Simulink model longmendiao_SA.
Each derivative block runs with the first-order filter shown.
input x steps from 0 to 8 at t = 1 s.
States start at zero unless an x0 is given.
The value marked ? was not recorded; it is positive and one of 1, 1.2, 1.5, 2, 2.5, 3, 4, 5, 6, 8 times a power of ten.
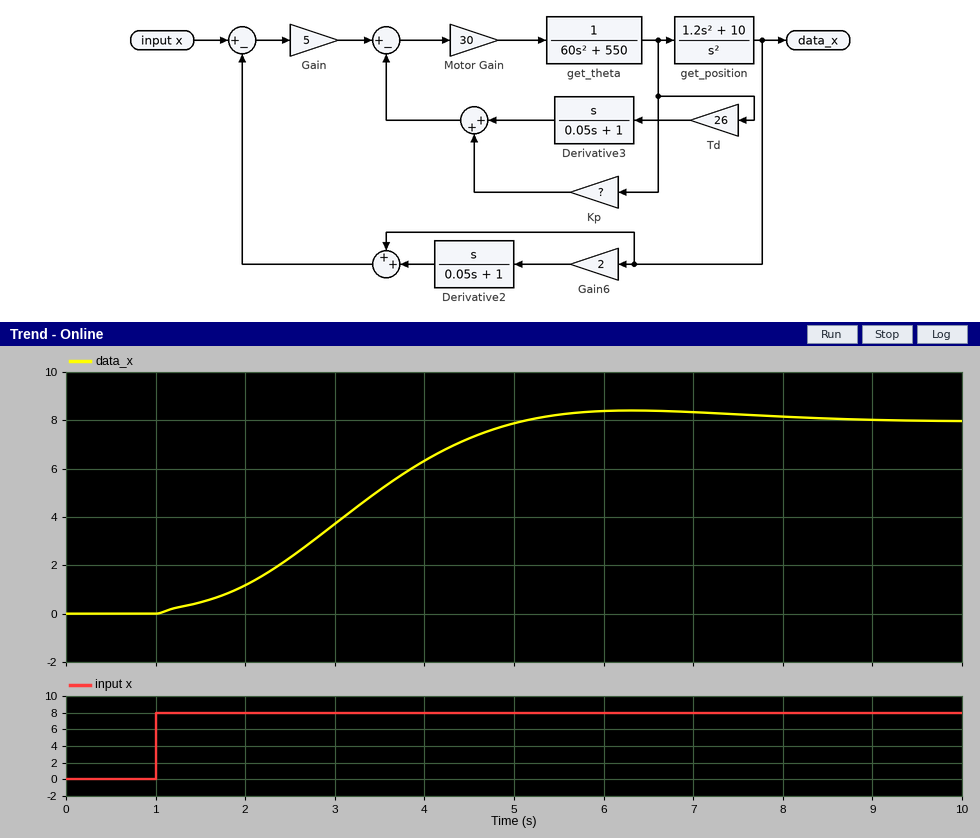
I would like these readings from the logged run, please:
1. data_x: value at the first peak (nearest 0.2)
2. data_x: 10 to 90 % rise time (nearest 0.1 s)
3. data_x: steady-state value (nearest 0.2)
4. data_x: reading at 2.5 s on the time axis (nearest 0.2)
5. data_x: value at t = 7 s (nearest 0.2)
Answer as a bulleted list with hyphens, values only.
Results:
- 8.4
- 2.7 s
- 8.0
- 2.4
- 8.4
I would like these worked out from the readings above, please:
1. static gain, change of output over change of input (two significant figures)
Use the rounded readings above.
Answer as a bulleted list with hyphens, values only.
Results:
- 1.0
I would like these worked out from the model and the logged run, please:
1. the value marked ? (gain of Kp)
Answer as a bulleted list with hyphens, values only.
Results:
- 80
